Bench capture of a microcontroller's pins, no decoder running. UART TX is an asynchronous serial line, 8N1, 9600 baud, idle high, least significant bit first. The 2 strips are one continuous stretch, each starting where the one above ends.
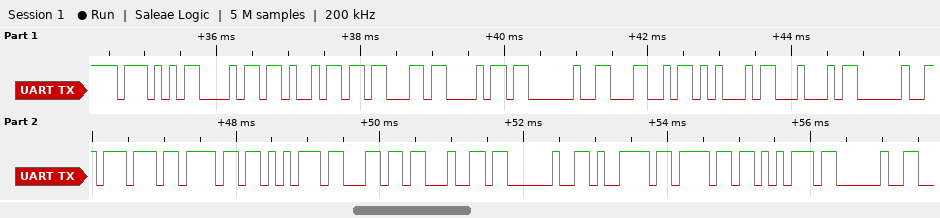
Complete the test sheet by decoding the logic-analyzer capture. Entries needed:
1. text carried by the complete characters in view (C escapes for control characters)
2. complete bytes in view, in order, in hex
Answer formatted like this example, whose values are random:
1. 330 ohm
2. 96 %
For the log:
1. "Which LED would you "
2. 57 68 69 63 68 20 4C 45 44 20 77 6F 75 6C 64 20 79 6F 75 20
